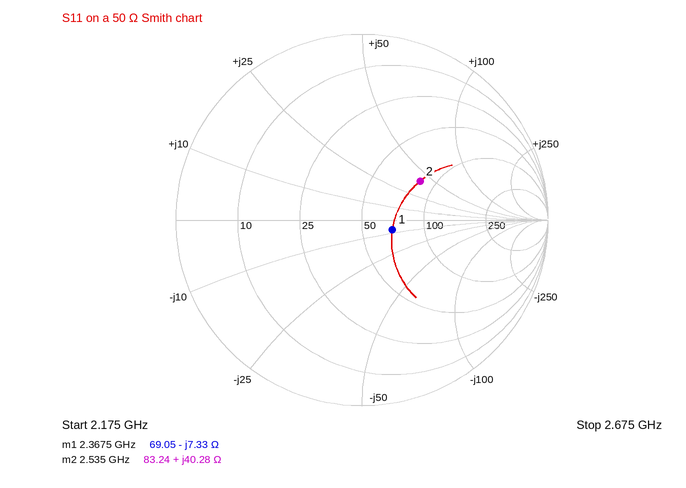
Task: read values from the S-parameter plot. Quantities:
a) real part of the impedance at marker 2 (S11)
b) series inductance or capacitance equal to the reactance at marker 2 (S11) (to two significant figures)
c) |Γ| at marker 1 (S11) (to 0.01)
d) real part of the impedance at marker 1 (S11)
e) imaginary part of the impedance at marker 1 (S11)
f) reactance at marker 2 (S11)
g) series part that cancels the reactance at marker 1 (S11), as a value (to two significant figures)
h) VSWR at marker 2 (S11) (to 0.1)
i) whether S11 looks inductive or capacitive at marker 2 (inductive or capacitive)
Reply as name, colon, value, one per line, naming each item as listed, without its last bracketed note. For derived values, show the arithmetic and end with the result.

real part of the impedance at marker 2: 83.24 Ω
series inductance or capacitance equal to the reactance at marker 2 (S11): L = 40.28 Ω/(2π × 2.535 GHz) ≈ 2.5 nH
|Γ| at marker 1 (S11): 0.17
real part of the impedance at marker 1: 69.05 Ω
imaginary part of the impedance at marker 1: -7.33 Ω
reactance at marker 2: +40.28 Ω
series part that cancels the reactance at marker 1 (S11), as a value: L = 7.33 Ω/(2π × 2.3675 GHz) ≈ 493 pH, so 490 pH to two significant figures
VSWR at marker 2 (S11): 2.2
whether S11 looks inductive or capacitive at marker 2: inductive
